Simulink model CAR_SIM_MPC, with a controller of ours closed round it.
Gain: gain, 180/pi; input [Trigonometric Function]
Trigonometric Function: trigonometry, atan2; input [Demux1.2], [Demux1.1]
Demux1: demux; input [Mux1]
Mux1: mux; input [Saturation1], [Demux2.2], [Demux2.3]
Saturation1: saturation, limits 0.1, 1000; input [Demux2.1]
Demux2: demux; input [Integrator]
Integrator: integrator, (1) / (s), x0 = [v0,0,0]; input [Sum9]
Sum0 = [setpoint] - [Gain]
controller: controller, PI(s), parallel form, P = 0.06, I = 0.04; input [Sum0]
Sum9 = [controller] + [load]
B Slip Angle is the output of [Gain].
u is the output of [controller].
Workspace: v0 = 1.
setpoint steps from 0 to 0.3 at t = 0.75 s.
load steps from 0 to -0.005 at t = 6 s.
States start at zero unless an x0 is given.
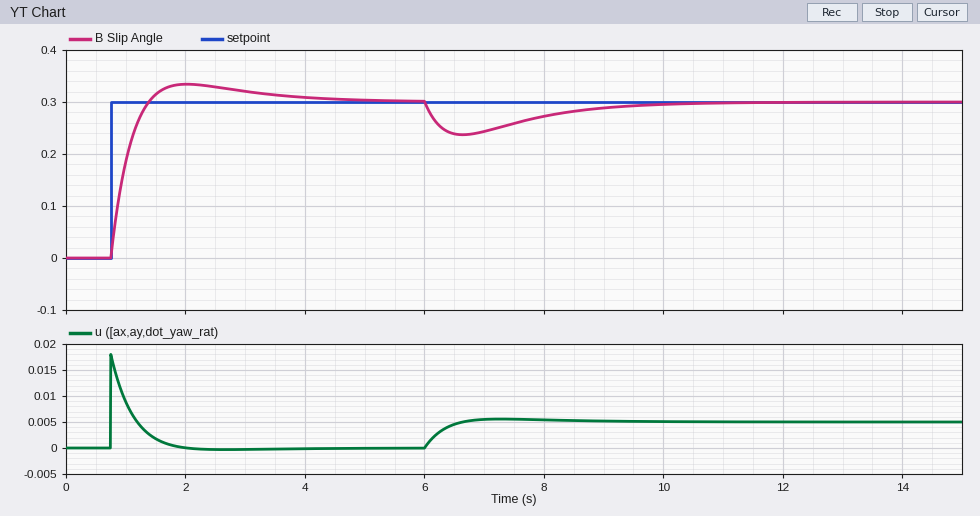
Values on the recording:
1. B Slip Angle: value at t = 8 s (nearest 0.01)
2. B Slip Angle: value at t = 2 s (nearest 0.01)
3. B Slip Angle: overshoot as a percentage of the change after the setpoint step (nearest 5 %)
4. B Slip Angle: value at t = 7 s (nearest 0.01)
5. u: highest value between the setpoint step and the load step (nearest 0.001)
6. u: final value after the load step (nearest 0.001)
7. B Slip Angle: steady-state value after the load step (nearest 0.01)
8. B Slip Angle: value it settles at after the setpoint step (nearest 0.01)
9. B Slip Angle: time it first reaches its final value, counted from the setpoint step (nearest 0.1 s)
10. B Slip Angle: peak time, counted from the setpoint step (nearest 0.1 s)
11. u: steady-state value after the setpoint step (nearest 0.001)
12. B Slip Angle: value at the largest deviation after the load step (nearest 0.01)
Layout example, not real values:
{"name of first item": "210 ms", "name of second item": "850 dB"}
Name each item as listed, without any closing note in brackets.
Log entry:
{"B Slip Angle: value at t = 8 s": "0.27", "B Slip Angle: value at t = 2 s": "0.33", "B Slip Angle: overshoot as a percentage of the change after the setpoint step": "10 %", "B Slip Angle: value at t = 7 s": "0.24", "u: highest value between the setpoint step and the load step": "0.018", "u: final value after the load step": "0.005", "B Slip Angle: steady-state value after the load step": "0.30", "B Slip Angle: value it settles at after the setpoint step": "0.30", "B Slip Angle: time it first reaches its final value, counted from the setpoint step": "0.6 s", "B Slip Angle: peak time, counted from the setpoint step": "1.3 s", "u: steady-state value after the setpoint step": "0.000", "B Slip Angle: value at the largest deviation after the load step": "0.24"}
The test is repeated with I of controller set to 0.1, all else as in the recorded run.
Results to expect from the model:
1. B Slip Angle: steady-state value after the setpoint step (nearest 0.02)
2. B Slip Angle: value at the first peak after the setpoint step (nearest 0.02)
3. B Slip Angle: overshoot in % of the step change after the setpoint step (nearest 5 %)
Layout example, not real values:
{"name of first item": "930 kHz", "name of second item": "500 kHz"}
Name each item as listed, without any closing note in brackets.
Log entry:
{"B Slip Angle: steady-state value after the setpoint step": "0.30", "B Slip Angle: value at the first peak after the setpoint step": "0.36", "B Slip Angle: overshoot in % of the step change after the setpoint step": "20 %"}
